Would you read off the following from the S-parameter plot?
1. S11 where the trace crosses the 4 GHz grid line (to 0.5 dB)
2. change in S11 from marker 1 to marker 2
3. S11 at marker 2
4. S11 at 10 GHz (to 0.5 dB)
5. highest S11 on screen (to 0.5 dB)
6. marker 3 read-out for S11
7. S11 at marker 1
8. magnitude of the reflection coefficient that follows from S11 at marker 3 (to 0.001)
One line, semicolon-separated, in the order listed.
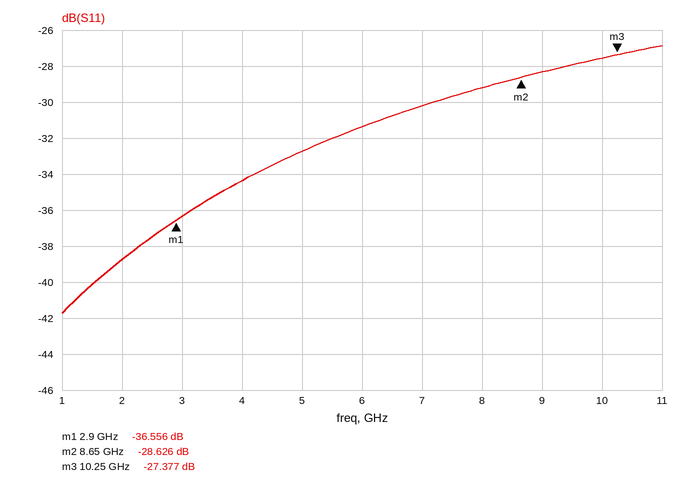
-34.5 dB; 7.930 dB; -28.626 dB; -27.5 dB; -27.0 dB; -27.377 dB; -36.556 dB; 0.043
